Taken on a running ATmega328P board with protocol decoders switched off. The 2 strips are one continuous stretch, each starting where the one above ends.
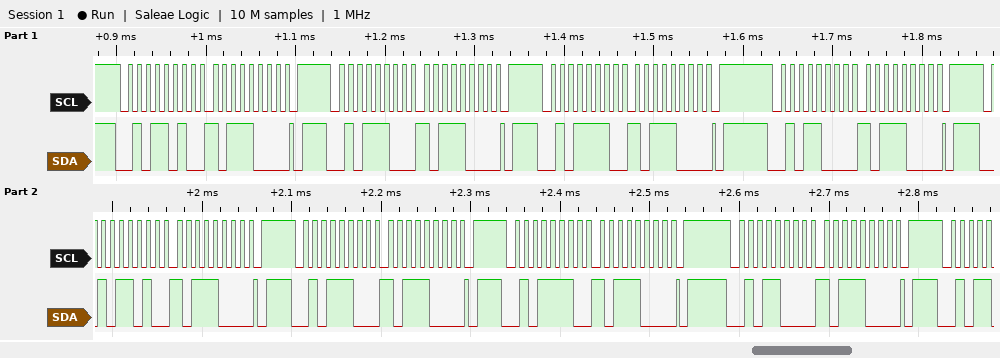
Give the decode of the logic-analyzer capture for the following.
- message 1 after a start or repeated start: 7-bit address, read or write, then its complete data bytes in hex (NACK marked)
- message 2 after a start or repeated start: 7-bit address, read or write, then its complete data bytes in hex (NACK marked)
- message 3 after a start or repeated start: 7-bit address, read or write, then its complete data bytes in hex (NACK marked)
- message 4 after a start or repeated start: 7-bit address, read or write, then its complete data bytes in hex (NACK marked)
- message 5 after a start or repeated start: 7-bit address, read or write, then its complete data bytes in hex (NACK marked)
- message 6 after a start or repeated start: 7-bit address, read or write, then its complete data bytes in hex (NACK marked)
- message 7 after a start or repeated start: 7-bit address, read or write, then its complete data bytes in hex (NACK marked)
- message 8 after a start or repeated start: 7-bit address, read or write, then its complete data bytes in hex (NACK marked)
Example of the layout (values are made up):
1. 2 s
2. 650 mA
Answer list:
1. 0x2D write: B8
2. 0x2E write: B8
3. 0x2F write: B8
4. 0x2C write: B8
5. 0x2D write: B8
6. 0x2E write: B8
7. 0x2F write: B8
8. 0x2C write: B8
